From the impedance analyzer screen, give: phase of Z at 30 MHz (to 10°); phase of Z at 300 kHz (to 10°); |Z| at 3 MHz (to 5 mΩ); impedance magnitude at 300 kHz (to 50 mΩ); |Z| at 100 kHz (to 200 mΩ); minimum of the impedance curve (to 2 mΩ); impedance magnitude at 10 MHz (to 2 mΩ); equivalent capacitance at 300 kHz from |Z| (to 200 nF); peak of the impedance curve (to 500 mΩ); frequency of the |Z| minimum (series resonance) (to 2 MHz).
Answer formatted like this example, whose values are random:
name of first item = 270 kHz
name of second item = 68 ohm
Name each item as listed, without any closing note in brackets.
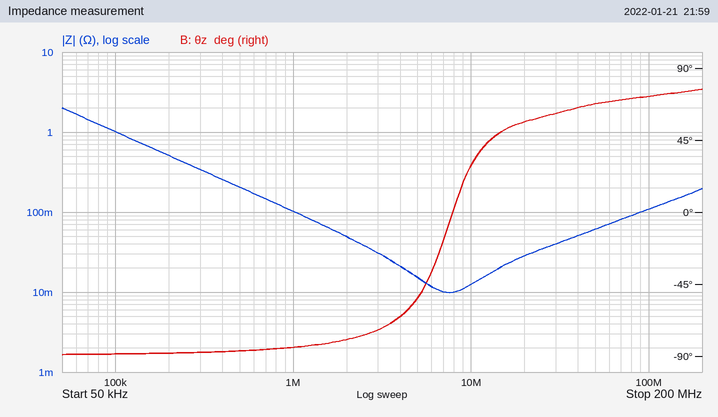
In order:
phase of Z at 30 MHz = 60°
phase of Z at 300 kHz = -90°
|Z| at 3 MHz = 30 mΩ
impedance magnitude at 300 kHz = 350 mΩ
|Z| at 100 kHz = 1.0 Ω
minimum of the impedance curve = 10 mΩ
impedance magnitude at 10 MHz = 12 mΩ
equivalent capacitance at 300 kHz from |Z| = 1.6 µF
peak of the impedance curve = 2.0 Ω
frequency of the |Z| minimum (series resonance) = 8 MHz
